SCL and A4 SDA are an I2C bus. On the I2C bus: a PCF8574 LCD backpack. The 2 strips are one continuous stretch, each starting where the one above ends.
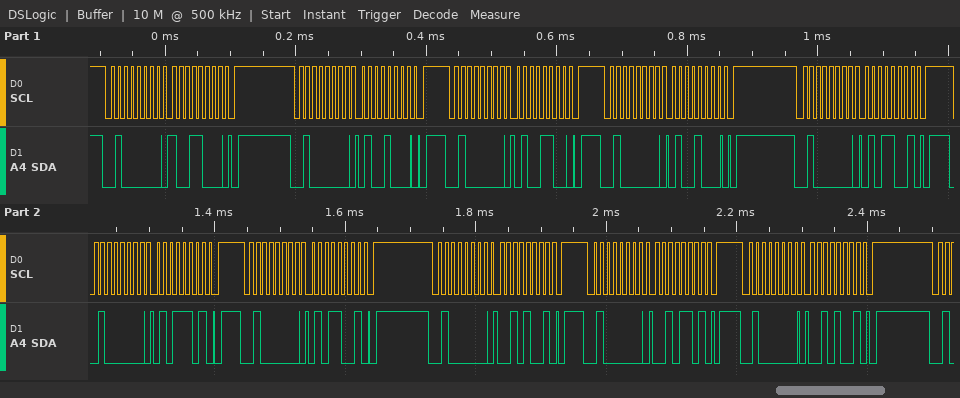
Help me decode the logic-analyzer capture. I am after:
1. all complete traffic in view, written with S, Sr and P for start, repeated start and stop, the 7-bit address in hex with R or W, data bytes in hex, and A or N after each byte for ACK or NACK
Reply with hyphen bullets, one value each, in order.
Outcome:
- S 20W A 98 A P S 20W A 48 A P S 20W A 4C A P S 20W A 48 A P S 20W A 59 A P S 20W A 5D A P S 20W A 59 A P S 20W A 29 A P S 20W A 2D A P S 20W A 29 A P
